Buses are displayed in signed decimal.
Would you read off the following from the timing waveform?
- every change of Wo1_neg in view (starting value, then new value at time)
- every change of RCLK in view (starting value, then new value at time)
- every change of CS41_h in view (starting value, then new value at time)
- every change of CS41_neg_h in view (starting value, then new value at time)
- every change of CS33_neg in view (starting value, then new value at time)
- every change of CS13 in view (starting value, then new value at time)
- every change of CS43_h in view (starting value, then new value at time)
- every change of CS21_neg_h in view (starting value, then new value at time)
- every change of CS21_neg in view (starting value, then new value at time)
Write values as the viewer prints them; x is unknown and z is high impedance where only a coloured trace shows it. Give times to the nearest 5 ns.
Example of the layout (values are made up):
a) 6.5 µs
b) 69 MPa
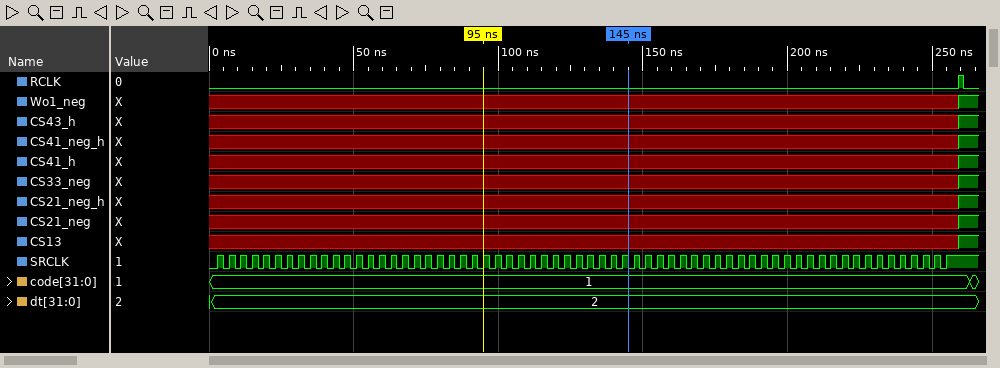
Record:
a) x, 1 at 260 ns
b) 0, 1 at 260 ns, 0 at 260 ns
c) x, 1 at 260 ns
d) x, 1 at 260 ns
e) x, 1 at 260 ns
f) x, 1 at 260 ns
g) x, 1 at 260 ns
h) x, 1 at 260 ns
i) x, 1 at 260 ns
